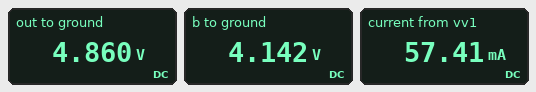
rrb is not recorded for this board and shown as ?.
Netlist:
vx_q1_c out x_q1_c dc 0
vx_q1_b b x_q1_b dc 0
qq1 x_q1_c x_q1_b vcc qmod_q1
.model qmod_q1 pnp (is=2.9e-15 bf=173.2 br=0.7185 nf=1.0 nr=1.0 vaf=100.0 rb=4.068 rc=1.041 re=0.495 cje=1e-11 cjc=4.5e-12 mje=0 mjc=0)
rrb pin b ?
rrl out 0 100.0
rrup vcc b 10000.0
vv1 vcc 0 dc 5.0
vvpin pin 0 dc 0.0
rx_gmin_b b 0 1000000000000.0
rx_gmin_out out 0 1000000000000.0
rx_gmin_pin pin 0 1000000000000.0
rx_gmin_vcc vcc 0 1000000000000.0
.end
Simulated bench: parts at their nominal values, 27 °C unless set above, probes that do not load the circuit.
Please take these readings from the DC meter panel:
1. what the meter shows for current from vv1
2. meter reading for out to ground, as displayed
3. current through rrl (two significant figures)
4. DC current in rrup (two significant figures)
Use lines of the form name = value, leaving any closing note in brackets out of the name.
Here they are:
what the meter shows for current from vv1 = 57.41 mA
meter reading for out to ground, as displayed = 4.860 V
current through rrl = 49 mA
DC current in rrup = 86 µA
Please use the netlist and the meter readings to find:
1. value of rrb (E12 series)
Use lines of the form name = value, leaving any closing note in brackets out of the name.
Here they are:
value of rrb = 470 Ω
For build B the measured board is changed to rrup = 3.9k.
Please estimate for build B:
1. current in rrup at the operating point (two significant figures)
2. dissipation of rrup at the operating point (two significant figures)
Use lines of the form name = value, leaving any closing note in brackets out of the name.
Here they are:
current in rrup at the operating point = 220 µA
dissipation of rrup at the operating point = 190 µW
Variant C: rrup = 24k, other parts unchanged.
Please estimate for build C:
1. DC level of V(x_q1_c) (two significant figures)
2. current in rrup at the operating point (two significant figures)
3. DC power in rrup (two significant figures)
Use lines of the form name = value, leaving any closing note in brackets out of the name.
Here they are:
DC level of V(x_q1_c) = 4.9 V
current in rrup at the operating point = 36 µA
DC power in rrup = 31 µW
